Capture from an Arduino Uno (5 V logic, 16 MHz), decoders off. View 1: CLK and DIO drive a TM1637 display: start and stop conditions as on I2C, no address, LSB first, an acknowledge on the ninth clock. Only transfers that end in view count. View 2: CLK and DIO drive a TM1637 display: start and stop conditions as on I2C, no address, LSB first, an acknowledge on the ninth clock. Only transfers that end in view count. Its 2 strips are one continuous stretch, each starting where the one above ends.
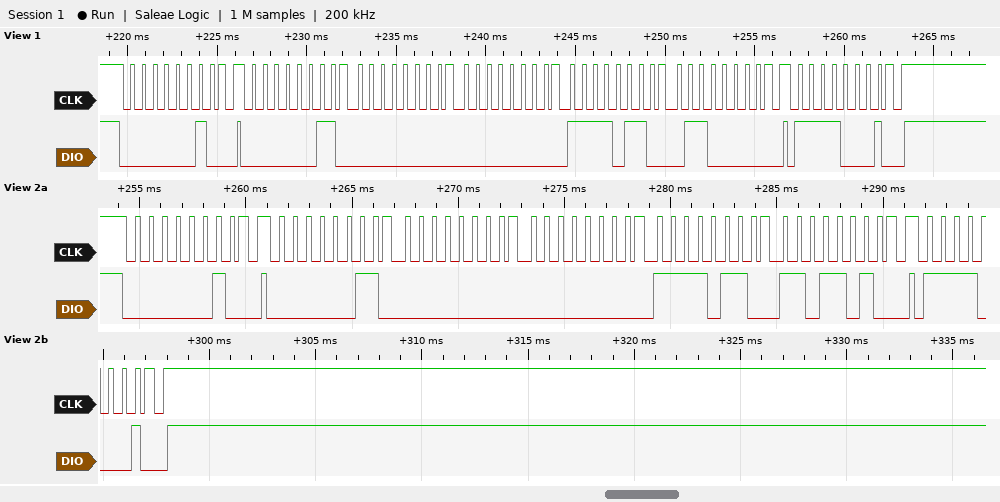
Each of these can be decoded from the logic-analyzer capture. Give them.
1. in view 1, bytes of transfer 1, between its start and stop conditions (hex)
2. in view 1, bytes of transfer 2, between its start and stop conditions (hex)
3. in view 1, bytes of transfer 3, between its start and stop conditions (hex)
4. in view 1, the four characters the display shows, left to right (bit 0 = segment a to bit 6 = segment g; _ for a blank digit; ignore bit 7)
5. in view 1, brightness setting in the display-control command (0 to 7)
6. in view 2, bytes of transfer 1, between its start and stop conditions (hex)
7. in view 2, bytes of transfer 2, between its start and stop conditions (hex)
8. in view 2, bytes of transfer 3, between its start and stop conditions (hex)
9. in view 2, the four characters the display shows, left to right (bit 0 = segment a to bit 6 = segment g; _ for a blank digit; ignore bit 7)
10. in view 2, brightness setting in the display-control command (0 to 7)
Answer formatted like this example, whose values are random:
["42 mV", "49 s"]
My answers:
["40", "C0 00 00 6F 06", "8F", "__91", "7", "40", "C0 00 00 6F 5B", "8F", "__92", "7"]
